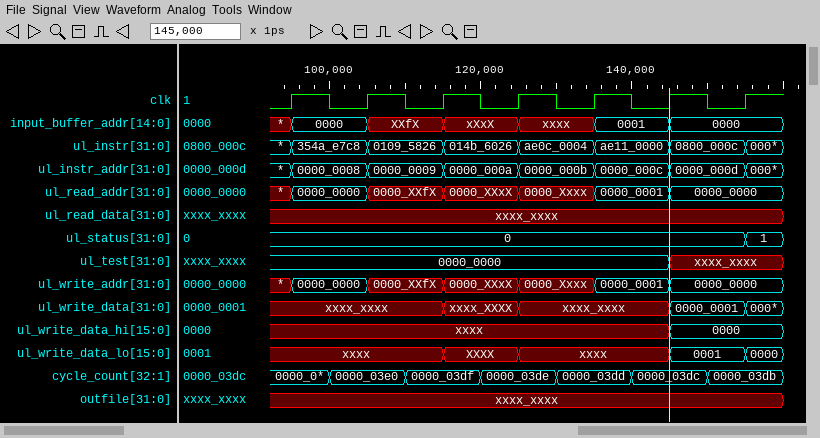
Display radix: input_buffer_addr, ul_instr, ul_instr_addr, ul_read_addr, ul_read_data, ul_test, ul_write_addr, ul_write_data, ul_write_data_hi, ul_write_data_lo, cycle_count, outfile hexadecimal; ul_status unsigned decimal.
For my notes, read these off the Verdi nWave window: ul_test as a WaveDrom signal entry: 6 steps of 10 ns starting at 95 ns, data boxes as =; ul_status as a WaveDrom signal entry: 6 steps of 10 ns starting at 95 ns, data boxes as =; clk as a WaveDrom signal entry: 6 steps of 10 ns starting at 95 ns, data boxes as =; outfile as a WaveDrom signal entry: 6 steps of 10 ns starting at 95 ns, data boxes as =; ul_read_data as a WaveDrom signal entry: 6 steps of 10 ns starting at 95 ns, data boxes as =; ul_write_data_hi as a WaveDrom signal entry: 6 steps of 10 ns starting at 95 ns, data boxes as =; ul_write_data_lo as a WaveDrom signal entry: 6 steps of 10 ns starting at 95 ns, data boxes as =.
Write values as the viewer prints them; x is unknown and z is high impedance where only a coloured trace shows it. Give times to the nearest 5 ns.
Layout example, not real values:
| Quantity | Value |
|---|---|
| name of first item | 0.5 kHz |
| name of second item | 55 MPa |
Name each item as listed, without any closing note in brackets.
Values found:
| Quantity | Value |
|---|---|
| ul_test as a WaveDrom signal entry: 6 steps of 10 ns starting at 95 ns, data boxes as = | {name: 'ul_test', wave: '=....x', data: '0000_0000'} |
| ul_status as a WaveDrom signal entry: 6 steps of 10 ns starting at 95 ns, data boxes as = | {name: 'ul_status', wave: '=.....', data: '0'} |
| clk as a WaveDrom signal entry: 6 steps of 10 ns starting at 95 ns, data boxes as = | {name: 'clk', wave: 'p.....'} |
| outfile as a WaveDrom signal entry: 6 steps of 10 ns starting at 95 ns, data boxes as = | {name: 'outfile', wave: 'x.....'} |
| ul_read_data as a WaveDrom signal entry: 6 steps of 10 ns starting at 95 ns, data boxes as = | {name: 'ul_read_data', wave: 'x.....'} |
| ul_write_data_hi as a WaveDrom signal entry: 6 steps of 10 ns starting at 95 ns, data boxes as = | {name: 'ul_write_data_hi', wave: 'x....=', data: '0000'} |
| ul_write_data_lo as a WaveDrom signal entry: 6 steps of 10 ns starting at 95 ns, data boxes as = | {name: 'ul_write_data_lo', wave: 'x.=x.=', data: 'XXXX 0001'} |
